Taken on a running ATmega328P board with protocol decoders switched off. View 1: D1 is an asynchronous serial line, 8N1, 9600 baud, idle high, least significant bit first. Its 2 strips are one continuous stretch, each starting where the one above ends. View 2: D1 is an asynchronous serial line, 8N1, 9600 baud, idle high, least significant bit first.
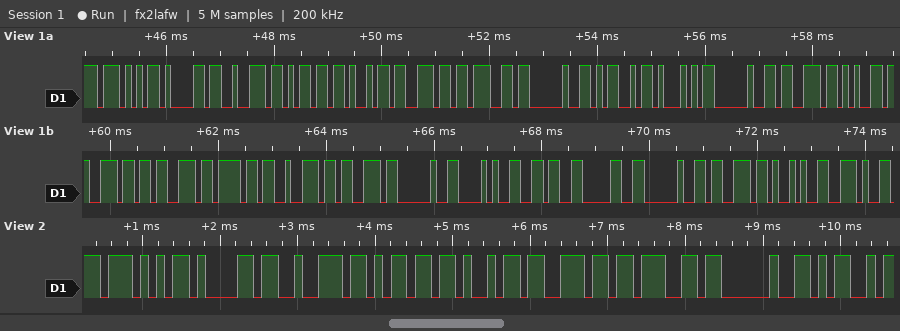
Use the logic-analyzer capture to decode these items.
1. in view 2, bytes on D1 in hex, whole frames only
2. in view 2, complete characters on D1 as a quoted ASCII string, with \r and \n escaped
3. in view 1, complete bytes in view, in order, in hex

57 61 72 6D 69 6E 67 20 4D
"Warming M"
57 61 72 6D 69 6E 67 20 4D 51 20 73 65 6E 73 6F 72 73 20 28 36 30 20 73 29 2E
